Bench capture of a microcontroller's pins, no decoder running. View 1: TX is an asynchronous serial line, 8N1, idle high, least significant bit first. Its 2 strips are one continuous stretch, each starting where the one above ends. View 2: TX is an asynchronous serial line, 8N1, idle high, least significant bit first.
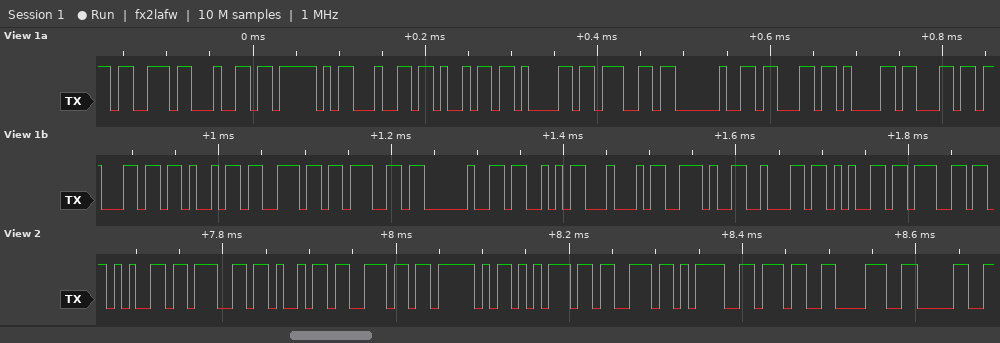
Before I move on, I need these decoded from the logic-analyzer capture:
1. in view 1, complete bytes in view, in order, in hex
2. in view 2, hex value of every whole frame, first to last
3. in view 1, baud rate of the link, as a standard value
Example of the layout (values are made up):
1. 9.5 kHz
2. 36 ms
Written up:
1. 73 64 5F 64 69 61 67 20 63 61 6C 6C 69 6E 67 20 53 44 2E 62 65 67
2. 65 67 69 6E 5F 75 73 3D 37 38 30
3. 115200 baud
